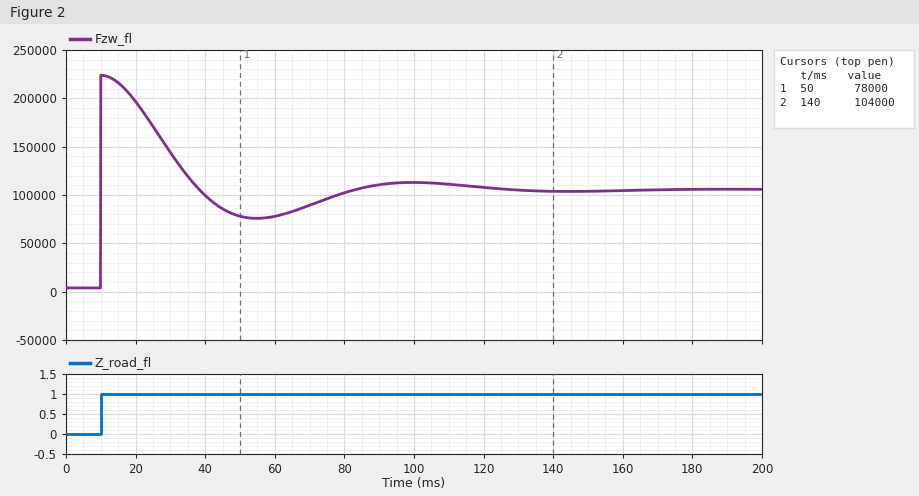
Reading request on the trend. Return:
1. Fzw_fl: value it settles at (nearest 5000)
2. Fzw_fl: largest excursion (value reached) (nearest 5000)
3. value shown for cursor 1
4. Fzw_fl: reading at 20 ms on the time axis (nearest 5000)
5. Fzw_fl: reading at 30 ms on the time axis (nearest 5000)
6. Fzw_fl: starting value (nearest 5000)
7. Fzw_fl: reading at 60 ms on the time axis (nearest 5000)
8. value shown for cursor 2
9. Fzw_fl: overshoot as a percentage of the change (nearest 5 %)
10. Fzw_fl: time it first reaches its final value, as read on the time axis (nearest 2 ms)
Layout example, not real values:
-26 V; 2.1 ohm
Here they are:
105000; 225000; 78000; 195000; 145000; 5000; 80000; 104000; 115 %; 10 ms
